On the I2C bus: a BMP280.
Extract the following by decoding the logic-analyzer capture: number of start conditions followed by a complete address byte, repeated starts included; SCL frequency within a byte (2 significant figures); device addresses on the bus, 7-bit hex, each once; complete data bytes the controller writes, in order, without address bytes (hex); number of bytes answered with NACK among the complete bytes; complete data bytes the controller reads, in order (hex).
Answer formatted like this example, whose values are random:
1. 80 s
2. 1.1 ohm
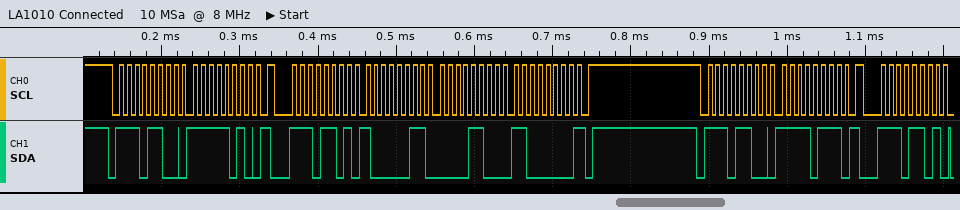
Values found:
1. 4
2. 100 kHz
3. 0x76
4. FA F7
5. 1
6. 83 0C C0
